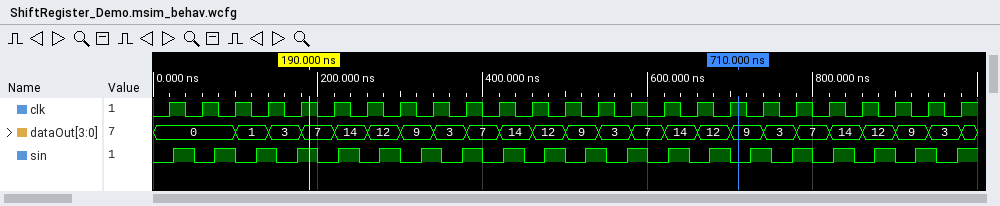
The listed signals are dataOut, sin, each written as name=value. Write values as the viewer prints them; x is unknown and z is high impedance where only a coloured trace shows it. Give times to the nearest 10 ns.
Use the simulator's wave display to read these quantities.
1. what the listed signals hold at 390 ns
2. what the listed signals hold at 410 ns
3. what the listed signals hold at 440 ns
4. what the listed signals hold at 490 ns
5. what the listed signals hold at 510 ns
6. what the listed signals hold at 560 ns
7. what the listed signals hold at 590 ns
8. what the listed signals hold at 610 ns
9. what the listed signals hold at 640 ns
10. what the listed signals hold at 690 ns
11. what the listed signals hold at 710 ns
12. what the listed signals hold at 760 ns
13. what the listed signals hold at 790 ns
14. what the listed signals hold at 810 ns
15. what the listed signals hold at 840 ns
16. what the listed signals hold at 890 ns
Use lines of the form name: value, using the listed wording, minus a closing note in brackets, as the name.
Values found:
what the listed signals hold at 390 ns: dataOut=7, sin=1
what the listed signals hold at 410 ns: dataOut=7, sin=0
what the listed signals hold at 440 ns: dataOut=14, sin=1
what the listed signals hold at 490 ns: dataOut=12, sin=1
what the listed signals hold at 510 ns: dataOut=9, sin=0
what the listed signals hold at 560 ns: dataOut=3, sin=0
what the listed signals hold at 590 ns: dataOut=7, sin=1
what the listed signals hold at 610 ns: dataOut=7, sin=0
what the listed signals hold at 640 ns: dataOut=14, sin=1
what the listed signals hold at 690 ns: dataOut=12, sin=1
what the listed signals hold at 710 ns: dataOut=9, sin=0
what the listed signals hold at 760 ns: dataOut=3, sin=0
what the listed signals hold at 790 ns: dataOut=7, sin=1
what the listed signals hold at 810 ns: dataOut=7, sin=0
what the listed signals hold at 840 ns: dataOut=14, sin=1
what the listed signals hold at 890 ns: dataOut=12, sin=1
